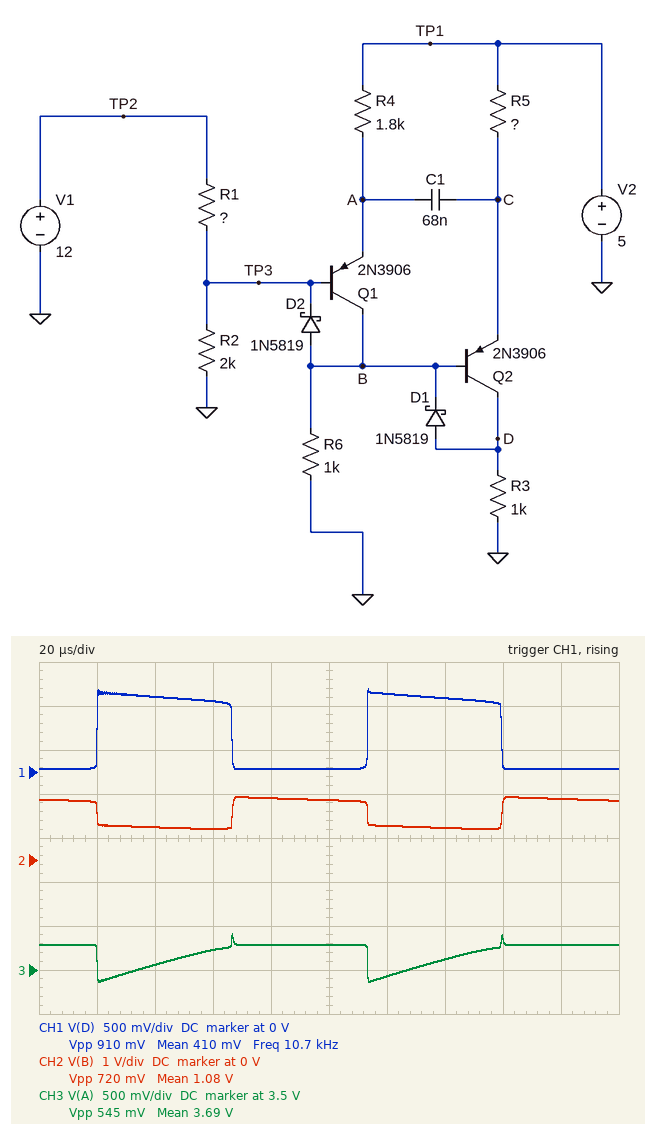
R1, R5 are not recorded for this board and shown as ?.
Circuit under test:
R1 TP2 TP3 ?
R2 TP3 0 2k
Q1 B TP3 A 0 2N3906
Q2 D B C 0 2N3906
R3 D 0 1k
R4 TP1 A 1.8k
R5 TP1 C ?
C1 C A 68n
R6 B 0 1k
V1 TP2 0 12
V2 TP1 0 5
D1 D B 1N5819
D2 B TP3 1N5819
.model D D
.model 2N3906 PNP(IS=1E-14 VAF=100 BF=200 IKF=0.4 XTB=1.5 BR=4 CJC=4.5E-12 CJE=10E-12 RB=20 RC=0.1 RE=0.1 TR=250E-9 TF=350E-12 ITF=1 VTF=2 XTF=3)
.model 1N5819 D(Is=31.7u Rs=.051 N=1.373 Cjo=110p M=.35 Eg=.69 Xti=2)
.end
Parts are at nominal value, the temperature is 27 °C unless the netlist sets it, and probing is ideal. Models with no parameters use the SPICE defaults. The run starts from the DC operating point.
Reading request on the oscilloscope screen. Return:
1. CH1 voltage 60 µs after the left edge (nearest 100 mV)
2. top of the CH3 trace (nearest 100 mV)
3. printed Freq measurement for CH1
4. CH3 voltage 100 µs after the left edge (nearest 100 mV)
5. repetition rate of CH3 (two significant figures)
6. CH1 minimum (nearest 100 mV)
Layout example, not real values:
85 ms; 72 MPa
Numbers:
800 mV; 3.9 V; 10.7 kHz; 3.8 V; 11 kHz; 0 V
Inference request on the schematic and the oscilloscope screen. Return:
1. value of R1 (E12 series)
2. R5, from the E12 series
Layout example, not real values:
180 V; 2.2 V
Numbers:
5.6 kΩ; 4.7 kΩ
